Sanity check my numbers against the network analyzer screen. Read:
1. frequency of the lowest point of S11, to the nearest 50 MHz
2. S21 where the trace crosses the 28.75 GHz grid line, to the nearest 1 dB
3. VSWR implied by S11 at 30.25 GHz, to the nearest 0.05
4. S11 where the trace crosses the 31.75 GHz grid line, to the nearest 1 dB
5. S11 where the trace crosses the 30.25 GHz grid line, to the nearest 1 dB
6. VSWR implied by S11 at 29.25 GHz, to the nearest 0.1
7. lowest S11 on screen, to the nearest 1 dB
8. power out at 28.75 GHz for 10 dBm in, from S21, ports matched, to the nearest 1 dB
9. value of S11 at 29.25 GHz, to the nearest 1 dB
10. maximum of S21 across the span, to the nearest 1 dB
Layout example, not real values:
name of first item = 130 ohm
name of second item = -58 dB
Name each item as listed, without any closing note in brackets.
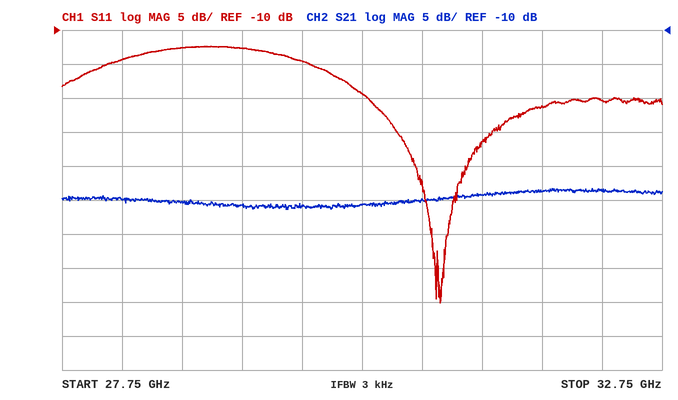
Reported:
frequency of the lowest point of S11, to the nearest 50 MHz = 30.90 GHz
S21 where the trace crosses the 28.75 GHz grid line, to the nearest 1 dB = -35 dB
VSWR implied by S11 at 30.25 GHz, to the nearest 0.05 = 1.25
S11 where the trace crosses the 31.75 GHz grid line, to the nearest 1 dB = -21 dB
S11 where the trace crosses the 30.25 GHz grid line, to the nearest 1 dB = -19 dB
VSWR implied by S11 at 29.25 GHz, to the nearest 0.1 = 1.6
lowest S11 on screen, to the nearest 1 dB = -50 dB
power out at 28.75 GHz for 10 dBm in, from S21, ports matched, to the nearest 1 dB = -25 dBm
value of S11 at 29.25 GHz, to the nearest 1 dB = -13 dB
maximum of S21 across the span, to the nearest 1 dB = -33 dB
